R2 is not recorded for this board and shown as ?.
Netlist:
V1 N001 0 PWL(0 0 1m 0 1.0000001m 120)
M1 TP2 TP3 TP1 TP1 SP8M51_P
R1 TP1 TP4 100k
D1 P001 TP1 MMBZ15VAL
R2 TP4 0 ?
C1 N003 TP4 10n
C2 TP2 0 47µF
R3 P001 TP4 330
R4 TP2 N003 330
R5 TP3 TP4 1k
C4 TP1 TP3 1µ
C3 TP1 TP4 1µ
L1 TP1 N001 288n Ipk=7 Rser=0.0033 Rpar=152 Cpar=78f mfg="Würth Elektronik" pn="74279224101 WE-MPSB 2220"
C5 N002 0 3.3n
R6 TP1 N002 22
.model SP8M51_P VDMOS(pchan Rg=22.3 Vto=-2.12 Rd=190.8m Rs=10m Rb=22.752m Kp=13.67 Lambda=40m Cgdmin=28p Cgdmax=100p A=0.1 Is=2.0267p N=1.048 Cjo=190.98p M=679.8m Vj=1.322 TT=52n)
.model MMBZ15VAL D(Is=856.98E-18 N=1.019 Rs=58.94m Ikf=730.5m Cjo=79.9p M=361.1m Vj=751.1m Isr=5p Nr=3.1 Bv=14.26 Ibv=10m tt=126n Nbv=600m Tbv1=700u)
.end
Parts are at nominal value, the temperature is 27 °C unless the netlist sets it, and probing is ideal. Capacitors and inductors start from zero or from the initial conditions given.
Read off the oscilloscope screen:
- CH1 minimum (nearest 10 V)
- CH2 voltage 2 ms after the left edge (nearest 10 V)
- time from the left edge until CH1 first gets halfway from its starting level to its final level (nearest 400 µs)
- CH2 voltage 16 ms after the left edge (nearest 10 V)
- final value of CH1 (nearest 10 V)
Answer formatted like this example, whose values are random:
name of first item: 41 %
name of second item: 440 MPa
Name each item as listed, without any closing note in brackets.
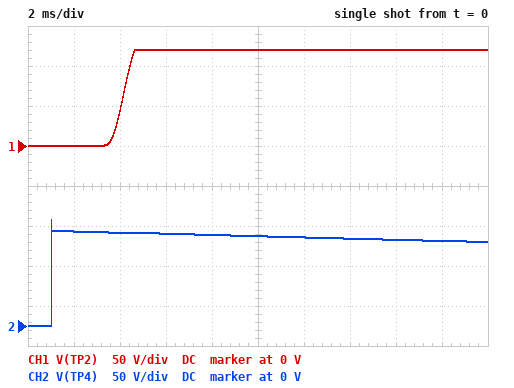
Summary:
CH1 minimum: 0 V
CH2 voltage 2 ms after the left edge: 120 V
time from the left edge until CH1 first gets halfway from its starting level to its final level: 4.0 ms
CH2 voltage 16 ms after the left edge: 110 V
final value of CH1: 120 V
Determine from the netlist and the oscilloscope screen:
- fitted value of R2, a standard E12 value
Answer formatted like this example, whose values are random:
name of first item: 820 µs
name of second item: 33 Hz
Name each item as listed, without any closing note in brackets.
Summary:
fitted value of R2, a standard E12 value: 68 kΩ
